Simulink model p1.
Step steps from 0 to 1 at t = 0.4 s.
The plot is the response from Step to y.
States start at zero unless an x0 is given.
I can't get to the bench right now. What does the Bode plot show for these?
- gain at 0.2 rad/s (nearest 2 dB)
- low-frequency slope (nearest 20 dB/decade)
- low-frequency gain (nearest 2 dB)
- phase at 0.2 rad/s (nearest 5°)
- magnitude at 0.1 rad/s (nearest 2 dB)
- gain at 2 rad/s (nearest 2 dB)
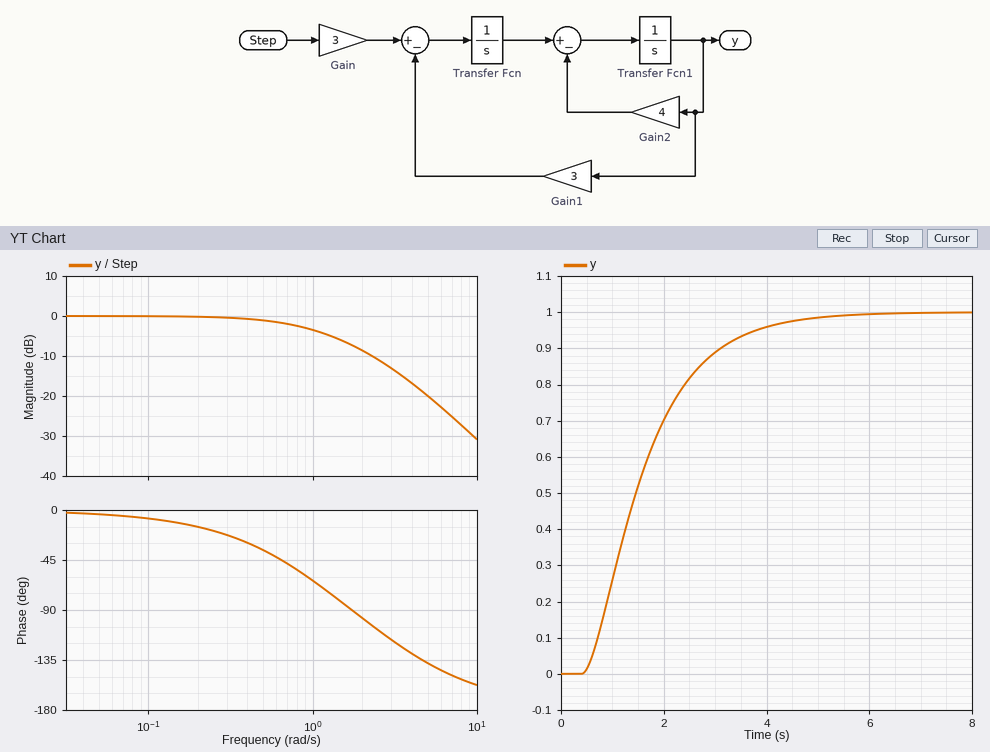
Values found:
0 dB
0 dB/decade
0 dB
-15°
0 dB
-8 dB
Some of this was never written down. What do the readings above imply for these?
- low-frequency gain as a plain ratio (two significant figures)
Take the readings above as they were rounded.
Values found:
1.0
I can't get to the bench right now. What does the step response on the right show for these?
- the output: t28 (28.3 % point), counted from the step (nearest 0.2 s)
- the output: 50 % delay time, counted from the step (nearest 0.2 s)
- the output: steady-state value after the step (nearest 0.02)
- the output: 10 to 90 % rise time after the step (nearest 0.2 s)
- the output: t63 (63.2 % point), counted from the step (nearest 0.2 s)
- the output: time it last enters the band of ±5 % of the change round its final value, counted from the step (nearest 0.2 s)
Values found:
0.6 s
1.0 s
1.00
2.4 s
1.4 s
3.4 s
